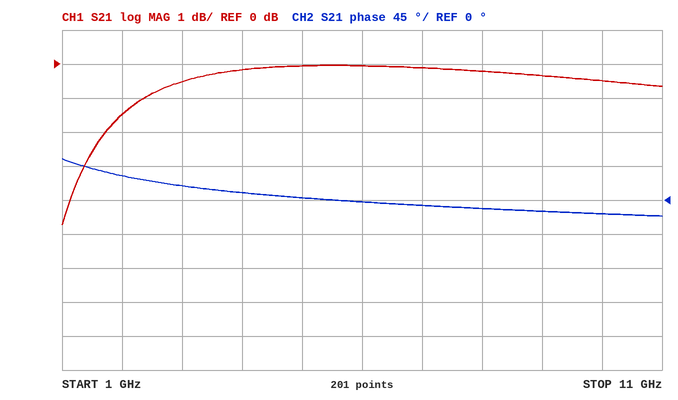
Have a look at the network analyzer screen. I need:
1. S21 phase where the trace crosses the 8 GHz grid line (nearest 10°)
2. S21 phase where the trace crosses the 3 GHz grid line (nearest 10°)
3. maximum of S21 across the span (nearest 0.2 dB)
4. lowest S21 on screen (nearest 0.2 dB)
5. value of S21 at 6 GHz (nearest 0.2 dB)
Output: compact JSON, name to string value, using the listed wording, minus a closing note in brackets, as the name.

{"S21 phase where the trace crosses the 8 GHz grid line": "-10°", "S21 phase where the trace crosses the 3 GHz grid line": "20°", "maximum of S21 across the span": "0.0 dB", "lowest S21 on screen": "-4.8 dB", "value of S21 at 6 GHz": "0.0 dB"}
